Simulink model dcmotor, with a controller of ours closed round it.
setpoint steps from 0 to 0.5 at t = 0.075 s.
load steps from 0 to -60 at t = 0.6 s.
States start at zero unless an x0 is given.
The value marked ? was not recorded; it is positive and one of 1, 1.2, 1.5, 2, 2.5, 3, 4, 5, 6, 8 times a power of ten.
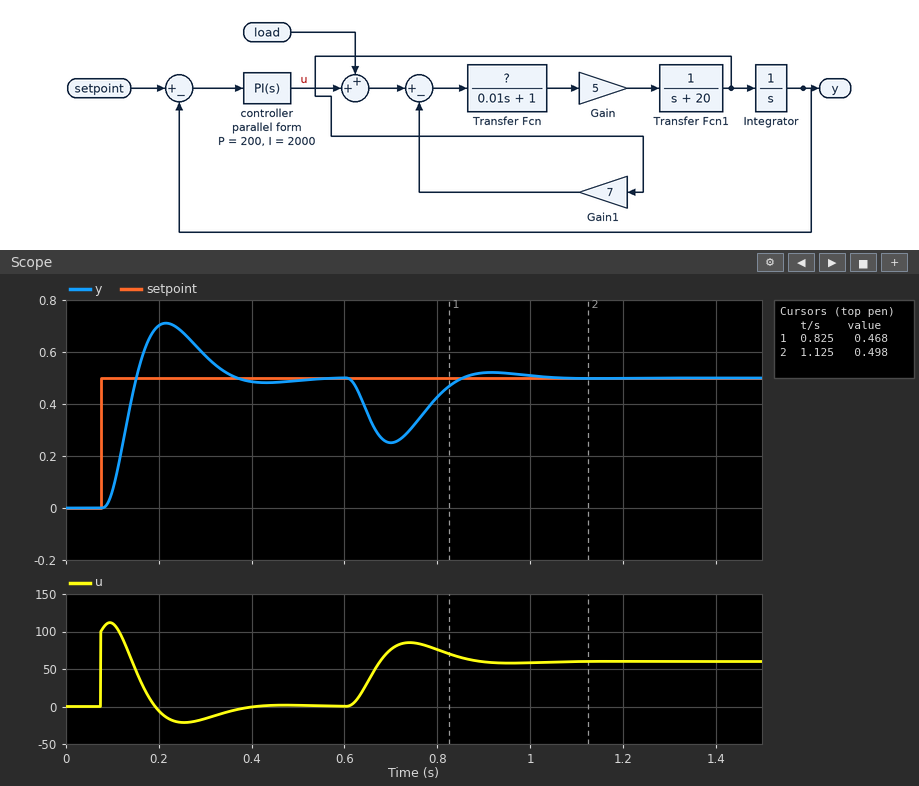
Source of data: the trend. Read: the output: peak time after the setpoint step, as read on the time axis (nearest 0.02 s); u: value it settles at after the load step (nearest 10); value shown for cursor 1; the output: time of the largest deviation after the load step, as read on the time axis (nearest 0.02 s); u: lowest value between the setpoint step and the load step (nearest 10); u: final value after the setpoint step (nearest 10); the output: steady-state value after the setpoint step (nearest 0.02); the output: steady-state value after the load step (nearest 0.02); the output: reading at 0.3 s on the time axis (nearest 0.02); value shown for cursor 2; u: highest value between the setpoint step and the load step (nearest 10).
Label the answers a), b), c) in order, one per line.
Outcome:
a) 0.22 s
b) 60
c) 0.468
d) 0.70 s
e) -20
f) 0
g) 0.50
h) 0.50
i) 0.58
j) 0.498
k) 110
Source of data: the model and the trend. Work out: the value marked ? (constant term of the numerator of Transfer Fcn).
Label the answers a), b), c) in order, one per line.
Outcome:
a) 1
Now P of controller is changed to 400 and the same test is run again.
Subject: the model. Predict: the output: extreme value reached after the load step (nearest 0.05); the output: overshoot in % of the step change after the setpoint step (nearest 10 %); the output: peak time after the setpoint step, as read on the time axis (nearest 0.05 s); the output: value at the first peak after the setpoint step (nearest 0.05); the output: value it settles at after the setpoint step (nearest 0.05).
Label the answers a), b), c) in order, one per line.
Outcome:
a) 0.35
b) 40 %
c) 0.15 s
d) 0.70
e) 0.50
